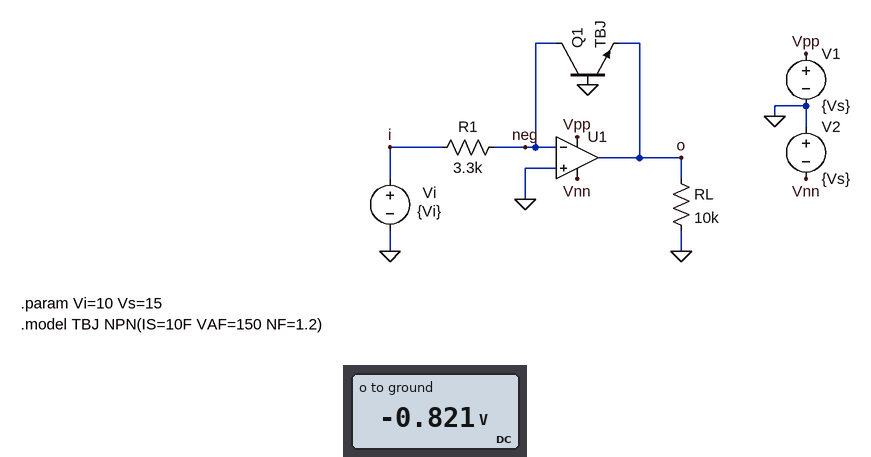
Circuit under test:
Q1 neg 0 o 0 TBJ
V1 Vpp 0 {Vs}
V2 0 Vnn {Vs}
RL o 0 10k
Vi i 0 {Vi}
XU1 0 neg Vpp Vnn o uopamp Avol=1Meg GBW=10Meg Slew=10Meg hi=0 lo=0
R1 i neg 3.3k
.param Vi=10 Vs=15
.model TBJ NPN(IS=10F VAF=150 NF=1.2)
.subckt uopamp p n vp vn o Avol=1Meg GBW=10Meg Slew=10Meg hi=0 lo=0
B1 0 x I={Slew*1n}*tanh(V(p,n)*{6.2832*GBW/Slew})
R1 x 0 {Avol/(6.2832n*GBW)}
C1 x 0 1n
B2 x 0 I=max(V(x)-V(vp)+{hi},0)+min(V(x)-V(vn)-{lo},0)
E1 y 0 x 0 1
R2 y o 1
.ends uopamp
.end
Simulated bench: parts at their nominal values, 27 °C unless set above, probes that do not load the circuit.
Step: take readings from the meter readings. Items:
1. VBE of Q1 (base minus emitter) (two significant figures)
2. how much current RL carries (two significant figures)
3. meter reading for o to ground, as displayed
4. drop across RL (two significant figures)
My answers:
820 mV
82 µA
-0.821 V
820 mV
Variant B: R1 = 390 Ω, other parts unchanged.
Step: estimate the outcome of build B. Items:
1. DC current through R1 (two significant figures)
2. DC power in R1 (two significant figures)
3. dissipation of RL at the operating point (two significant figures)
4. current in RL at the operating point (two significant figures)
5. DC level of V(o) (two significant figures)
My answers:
26 mA
260 mW
79 µW
89 µA
-890 mV
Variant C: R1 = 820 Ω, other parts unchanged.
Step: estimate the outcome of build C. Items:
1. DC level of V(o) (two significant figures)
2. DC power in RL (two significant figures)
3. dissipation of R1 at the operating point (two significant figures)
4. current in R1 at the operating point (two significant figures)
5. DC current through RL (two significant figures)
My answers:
-860 mV
75 µW
120 mW
12 mA
86 µA
